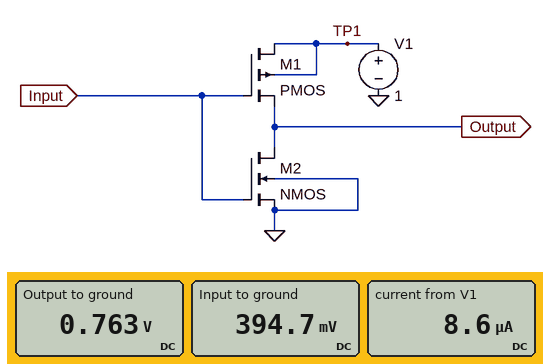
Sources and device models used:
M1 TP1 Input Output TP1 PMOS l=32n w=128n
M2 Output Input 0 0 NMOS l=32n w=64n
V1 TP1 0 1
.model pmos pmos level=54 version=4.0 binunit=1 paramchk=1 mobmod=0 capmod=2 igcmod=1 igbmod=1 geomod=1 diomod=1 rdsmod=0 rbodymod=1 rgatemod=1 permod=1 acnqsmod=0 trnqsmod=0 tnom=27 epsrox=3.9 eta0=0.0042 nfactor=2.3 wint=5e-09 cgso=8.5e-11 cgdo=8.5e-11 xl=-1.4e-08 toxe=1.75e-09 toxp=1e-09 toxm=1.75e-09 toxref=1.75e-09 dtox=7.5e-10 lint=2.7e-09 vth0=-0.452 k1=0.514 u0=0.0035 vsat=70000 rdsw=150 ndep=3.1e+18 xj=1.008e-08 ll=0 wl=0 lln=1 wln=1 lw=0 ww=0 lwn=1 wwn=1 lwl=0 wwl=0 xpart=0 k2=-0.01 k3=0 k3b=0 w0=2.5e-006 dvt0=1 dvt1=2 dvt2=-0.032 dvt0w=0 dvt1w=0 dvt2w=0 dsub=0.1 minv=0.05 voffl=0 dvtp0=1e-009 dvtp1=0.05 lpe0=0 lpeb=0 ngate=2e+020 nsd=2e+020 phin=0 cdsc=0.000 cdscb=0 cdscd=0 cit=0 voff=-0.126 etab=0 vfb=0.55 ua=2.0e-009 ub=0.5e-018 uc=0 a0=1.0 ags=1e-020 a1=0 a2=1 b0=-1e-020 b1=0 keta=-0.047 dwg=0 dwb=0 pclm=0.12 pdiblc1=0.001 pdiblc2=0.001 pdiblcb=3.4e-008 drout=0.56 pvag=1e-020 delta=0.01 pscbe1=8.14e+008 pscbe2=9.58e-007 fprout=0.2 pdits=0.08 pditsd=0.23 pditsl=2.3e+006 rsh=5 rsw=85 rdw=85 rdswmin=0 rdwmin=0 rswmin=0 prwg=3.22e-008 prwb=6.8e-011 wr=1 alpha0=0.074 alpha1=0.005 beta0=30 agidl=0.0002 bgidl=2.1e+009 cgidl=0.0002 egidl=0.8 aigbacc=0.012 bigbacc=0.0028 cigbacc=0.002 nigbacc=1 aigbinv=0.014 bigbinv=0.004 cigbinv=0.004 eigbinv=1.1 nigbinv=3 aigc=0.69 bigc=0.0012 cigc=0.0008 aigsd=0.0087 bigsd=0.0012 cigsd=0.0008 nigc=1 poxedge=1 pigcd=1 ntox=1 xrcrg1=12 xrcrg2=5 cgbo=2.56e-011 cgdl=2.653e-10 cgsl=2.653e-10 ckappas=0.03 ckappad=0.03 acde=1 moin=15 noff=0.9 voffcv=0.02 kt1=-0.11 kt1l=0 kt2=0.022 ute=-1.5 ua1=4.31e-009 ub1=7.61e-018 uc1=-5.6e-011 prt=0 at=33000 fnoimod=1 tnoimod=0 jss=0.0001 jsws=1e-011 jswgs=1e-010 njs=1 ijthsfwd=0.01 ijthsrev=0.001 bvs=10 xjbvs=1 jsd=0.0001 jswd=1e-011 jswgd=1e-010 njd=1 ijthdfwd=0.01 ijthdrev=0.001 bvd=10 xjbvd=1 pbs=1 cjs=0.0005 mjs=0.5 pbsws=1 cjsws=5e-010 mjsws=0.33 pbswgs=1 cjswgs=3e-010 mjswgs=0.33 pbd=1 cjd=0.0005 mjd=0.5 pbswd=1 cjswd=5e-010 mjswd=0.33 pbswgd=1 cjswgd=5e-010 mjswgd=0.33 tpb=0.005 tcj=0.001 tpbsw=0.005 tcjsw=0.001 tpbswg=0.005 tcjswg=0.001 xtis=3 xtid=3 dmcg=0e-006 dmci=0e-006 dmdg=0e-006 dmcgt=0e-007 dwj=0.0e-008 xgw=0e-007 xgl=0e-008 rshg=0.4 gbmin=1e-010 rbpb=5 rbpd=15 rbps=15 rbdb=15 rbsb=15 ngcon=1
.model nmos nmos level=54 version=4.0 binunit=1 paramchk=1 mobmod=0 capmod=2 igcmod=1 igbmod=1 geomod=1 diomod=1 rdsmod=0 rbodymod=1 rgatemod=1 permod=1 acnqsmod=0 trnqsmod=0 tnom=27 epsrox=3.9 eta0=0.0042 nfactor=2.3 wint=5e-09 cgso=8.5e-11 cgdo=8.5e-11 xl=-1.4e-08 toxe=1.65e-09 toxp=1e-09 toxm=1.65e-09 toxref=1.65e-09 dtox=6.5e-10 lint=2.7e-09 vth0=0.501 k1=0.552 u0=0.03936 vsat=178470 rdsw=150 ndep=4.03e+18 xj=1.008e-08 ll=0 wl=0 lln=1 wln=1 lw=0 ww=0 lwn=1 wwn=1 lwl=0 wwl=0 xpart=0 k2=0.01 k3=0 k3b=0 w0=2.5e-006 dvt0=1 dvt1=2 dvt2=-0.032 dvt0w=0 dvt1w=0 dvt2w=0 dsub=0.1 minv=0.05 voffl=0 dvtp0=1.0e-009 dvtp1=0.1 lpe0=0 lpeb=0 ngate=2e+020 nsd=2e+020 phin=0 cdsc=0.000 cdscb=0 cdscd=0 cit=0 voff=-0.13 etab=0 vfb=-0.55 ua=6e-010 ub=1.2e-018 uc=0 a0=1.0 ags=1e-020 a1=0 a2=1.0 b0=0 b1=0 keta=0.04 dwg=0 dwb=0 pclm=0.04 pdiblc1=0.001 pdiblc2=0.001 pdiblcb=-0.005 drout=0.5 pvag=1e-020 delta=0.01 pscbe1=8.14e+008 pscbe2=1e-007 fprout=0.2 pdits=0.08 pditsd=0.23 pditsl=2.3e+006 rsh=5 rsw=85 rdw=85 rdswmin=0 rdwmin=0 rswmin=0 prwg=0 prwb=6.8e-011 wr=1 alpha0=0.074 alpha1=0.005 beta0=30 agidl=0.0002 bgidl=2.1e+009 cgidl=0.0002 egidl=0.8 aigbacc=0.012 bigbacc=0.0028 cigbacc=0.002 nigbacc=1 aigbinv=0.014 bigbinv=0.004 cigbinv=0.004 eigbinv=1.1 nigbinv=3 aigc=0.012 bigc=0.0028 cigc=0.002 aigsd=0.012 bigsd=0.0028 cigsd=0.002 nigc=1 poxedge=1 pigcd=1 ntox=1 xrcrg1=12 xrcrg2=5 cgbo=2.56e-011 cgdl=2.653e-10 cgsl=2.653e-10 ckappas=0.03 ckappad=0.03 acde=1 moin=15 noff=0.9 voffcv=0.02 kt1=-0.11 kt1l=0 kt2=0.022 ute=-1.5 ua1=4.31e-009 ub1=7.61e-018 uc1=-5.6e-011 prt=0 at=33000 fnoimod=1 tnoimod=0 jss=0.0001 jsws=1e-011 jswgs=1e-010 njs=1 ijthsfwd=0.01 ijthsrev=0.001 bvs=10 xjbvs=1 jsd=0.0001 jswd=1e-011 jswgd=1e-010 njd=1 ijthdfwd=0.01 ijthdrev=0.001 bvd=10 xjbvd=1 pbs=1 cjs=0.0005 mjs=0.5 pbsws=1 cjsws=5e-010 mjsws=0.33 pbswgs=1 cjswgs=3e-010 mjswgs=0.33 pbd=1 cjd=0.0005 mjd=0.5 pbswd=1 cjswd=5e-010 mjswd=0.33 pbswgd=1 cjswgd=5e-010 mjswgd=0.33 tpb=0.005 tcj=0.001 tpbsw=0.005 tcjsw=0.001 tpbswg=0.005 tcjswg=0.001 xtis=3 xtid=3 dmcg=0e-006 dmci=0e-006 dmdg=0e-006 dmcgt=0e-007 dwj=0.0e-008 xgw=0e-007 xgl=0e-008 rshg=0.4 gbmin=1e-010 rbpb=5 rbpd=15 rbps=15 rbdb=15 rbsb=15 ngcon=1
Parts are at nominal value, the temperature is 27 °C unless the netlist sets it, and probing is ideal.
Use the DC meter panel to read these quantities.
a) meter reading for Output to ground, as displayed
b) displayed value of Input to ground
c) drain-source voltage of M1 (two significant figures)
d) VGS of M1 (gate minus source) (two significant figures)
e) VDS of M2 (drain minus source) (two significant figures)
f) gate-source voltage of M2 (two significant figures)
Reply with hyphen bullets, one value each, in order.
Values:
- 0.763 V
- 394.7 mV
- 240 mV
- -370 mV
- 760 mV
- 390 mV
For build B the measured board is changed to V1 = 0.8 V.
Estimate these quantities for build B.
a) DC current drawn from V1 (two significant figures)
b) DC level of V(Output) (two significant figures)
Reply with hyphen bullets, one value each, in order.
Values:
- 2.1 µA
- 620 mV
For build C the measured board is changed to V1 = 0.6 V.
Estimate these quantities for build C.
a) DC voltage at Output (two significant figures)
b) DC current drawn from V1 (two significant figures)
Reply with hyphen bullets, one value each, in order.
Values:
- 460 mV
- 230 nA
